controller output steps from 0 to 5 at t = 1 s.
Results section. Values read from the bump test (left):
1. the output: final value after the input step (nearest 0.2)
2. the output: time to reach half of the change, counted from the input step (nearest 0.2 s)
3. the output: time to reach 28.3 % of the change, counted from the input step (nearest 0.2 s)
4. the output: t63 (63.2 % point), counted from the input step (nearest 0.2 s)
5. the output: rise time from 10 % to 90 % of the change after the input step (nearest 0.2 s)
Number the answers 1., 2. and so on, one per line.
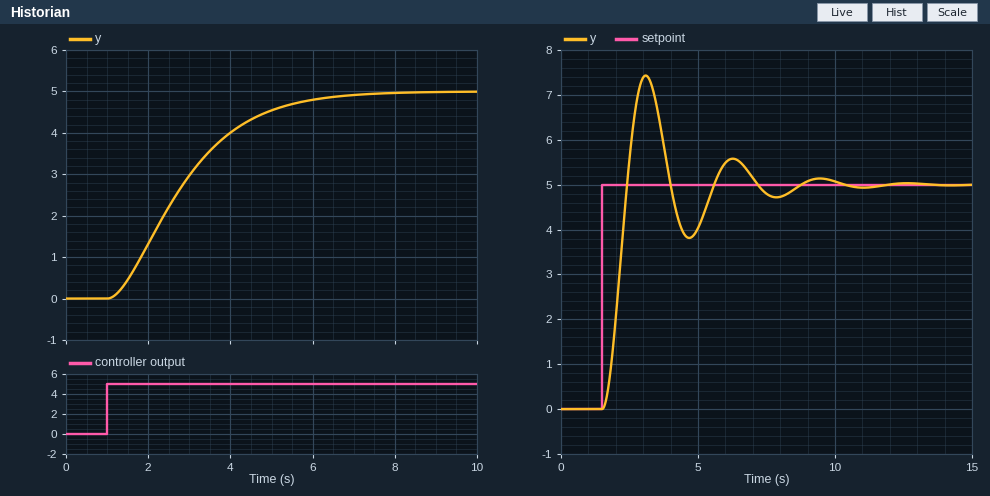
1. 5.0
2. 1.6 s
3. 1.0 s
4. 2.2 s
5. 3.4 s
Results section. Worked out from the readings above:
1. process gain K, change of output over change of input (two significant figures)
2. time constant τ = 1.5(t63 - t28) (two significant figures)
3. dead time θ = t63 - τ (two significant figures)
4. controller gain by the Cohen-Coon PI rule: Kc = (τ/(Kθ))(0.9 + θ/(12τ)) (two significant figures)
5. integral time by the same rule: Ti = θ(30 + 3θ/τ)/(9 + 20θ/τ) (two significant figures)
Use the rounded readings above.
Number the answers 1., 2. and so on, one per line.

1. 1.0
2. 1.8 s
3. 0.40 s
4. 4.1
5. 0.91 s
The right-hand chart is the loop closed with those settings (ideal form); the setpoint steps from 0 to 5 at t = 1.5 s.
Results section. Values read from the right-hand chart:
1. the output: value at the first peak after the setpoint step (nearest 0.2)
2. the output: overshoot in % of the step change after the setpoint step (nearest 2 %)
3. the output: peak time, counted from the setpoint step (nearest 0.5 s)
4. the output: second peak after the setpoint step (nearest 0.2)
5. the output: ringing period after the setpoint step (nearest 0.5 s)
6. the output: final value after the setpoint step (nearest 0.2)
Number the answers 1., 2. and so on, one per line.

1. 7.4
2. 48 %
3. 1.5 s
4. 5.6
5. 3.0 s
6. 5.0
